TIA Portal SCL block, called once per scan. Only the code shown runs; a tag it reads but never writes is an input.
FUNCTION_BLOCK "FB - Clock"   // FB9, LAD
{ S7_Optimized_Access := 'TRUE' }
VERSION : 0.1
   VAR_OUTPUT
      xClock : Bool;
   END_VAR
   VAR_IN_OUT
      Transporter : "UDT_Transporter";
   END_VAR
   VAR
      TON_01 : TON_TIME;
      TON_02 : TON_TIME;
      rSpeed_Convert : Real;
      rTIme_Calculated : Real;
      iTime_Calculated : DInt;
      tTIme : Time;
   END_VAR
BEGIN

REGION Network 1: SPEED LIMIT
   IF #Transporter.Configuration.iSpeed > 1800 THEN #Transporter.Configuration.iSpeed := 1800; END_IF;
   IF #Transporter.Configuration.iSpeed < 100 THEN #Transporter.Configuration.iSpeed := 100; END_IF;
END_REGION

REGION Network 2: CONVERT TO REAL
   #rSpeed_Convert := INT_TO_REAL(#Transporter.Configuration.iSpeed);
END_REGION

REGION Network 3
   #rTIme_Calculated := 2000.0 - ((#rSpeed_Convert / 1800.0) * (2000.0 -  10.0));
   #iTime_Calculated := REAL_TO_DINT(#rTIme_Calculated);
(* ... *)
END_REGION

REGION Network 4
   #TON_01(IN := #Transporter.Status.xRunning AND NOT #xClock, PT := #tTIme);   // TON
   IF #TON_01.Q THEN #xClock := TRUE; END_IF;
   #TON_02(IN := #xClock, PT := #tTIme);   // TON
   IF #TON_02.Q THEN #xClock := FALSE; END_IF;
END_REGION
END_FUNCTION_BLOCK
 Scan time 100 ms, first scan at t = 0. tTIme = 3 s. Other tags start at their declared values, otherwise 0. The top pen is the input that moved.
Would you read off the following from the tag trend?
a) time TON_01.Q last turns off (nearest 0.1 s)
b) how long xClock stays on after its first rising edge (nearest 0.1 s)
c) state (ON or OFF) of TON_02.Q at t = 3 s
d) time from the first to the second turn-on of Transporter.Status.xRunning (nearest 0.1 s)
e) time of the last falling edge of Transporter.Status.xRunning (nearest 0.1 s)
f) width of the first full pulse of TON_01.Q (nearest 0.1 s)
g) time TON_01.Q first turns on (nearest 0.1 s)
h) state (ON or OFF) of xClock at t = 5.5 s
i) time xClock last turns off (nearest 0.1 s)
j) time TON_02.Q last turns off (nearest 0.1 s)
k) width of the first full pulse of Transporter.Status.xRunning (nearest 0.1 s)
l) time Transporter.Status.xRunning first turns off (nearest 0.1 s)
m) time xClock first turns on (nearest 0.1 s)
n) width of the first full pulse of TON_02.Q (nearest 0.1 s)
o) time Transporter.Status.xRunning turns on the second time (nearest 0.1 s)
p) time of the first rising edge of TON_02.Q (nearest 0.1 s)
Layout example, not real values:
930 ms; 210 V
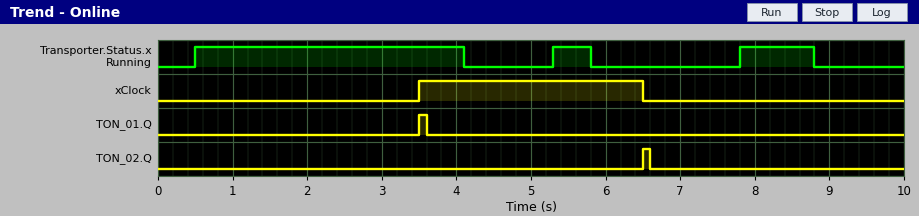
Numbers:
3.6 s; 3.0 s; OFF; 4.8 s; 8.8 s; 0.1 s; 3.5 s; ON; 6.5 s; 6.6 s; 3.6 s; 4.1 s; 3.5 s; 0.1 s; 5.3 s; 6.5 s
